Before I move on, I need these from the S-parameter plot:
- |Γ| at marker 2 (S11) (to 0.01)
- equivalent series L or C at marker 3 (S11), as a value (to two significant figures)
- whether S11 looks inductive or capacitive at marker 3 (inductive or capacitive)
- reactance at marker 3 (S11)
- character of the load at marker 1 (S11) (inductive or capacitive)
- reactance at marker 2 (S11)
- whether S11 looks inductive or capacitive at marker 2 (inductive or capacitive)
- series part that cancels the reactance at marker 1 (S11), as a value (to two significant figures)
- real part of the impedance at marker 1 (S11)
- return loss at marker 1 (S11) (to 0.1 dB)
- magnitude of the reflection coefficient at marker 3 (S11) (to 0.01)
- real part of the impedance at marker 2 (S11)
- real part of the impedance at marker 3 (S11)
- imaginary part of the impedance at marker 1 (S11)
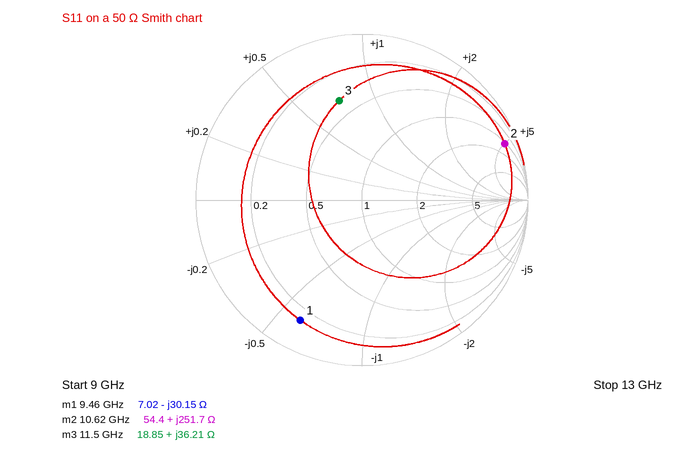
0.92
500 pH
inductive
+36.21 Ω
capacitive
+251.7 Ω
inductive
510 pH
7.02 Ω
1.8 dB
0.61
54.4 Ω
18.85 Ω
-30.15 Ω
